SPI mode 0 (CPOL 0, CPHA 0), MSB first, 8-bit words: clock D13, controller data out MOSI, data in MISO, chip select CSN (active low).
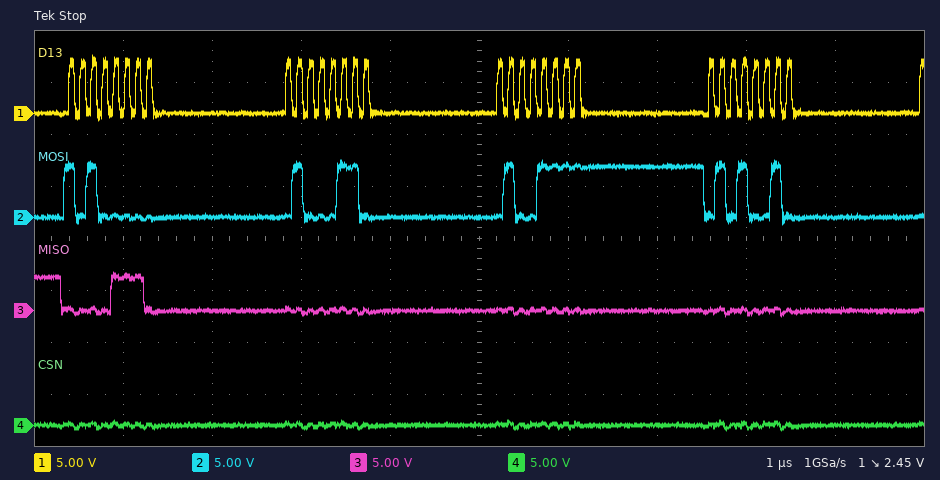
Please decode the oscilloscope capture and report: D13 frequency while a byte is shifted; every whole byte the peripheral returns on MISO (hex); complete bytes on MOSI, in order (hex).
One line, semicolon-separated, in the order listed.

8 MHz; 0E 00 00 00; A0 46 4F 52
